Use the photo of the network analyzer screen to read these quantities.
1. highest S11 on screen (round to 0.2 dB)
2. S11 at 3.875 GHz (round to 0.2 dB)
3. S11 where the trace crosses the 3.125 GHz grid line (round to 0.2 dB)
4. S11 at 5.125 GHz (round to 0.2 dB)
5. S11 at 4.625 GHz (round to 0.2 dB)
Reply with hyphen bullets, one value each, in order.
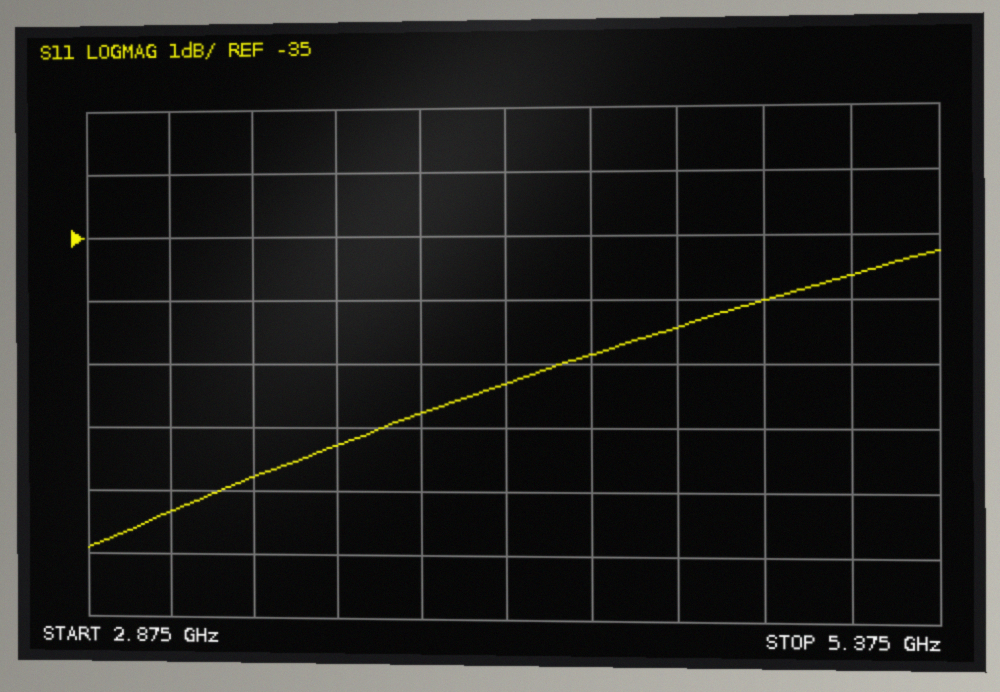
- -35.2 dB
- -37.8 dB
- -39.4 dB
- -35.6 dB
- -36.4 dB
